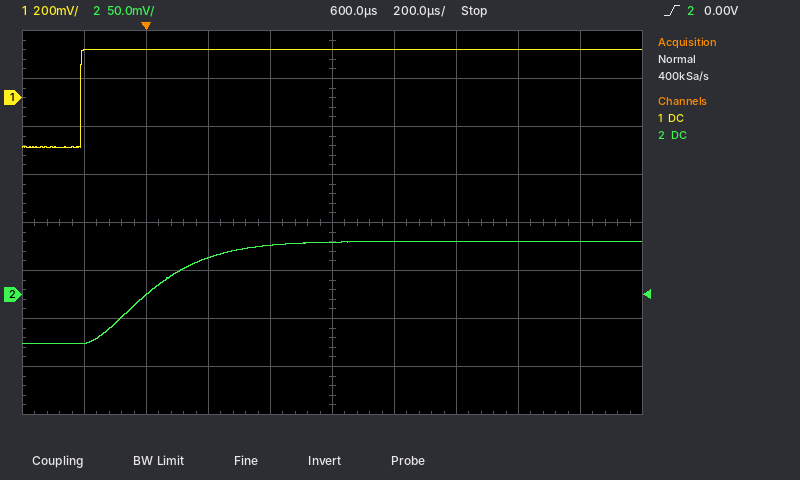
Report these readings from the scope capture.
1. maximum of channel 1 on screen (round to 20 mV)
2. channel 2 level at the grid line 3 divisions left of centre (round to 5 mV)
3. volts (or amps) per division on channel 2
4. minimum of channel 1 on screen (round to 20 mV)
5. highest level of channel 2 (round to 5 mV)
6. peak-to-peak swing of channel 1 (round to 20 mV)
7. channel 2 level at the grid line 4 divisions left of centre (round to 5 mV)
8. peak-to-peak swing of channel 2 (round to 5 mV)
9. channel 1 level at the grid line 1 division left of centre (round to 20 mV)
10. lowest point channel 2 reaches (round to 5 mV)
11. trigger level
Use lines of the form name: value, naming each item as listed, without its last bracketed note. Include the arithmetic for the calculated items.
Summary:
maximum of channel 1 on screen: 200 mV
channel 2 level at the grid line 3 divisions left of centre: 0 mV
volts (or amps) per division on channel 2: 50 mV
minimum of channel 1 on screen: -200 mV
highest level of channel 2: 55 mV
peak-to-peak swing of channel 1: 200 mV − (-200 mV) = 400 mV
channel 2 level at the grid line 4 divisions left of centre: -50 mV
peak-to-peak swing of channel 2: 55 mV − (-50 mV) = 105 mV
channel 1 level at the grid line 1 division left of centre: 200 mV
lowest point channel 2 reaches: -50 mV
trigger level: 0.00 V
